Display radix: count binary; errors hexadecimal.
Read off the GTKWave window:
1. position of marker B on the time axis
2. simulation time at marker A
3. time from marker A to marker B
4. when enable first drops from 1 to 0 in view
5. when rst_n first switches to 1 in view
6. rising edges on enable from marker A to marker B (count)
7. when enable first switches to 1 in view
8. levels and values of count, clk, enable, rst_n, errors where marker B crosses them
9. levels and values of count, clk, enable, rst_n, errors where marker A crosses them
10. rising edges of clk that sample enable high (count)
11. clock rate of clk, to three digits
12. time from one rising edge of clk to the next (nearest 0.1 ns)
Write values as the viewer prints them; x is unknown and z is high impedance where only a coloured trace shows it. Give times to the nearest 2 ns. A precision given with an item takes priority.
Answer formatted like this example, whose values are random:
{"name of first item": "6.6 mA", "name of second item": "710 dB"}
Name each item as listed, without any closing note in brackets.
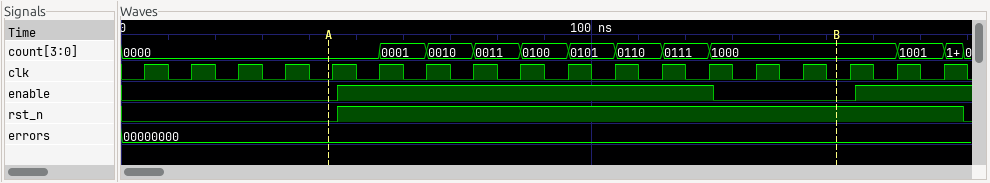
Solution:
{"position of marker B on the time axis": "152 ns", "simulation time at marker A": "44 ns", "time from marker A to marker B": "108 ns", "when enable first drops from 1 to 0 in view": "126 ns", "when rst_n first switches to 1 in view": "46 ns", "rising edges on enable from marker A to marker B": "1", "when enable first switches to 1 in view": "46 ns", "levels and values of count, clk, enable, rst_n, errors where marker B crosses them": "count=1000, clk=0, enable=0, rst_n=1, errors=00000000", "levels and values of count, clk, enable, rst_n, errors where marker A crosses them": "count=0000, clk=0, enable=0, rst_n=0, errors=00000000", "rising edges of clk that sample enable high": "10", "clock rate of clk, to three digits": "100 MHz", "time from one rising edge of clk to the next": "10 ns"}
